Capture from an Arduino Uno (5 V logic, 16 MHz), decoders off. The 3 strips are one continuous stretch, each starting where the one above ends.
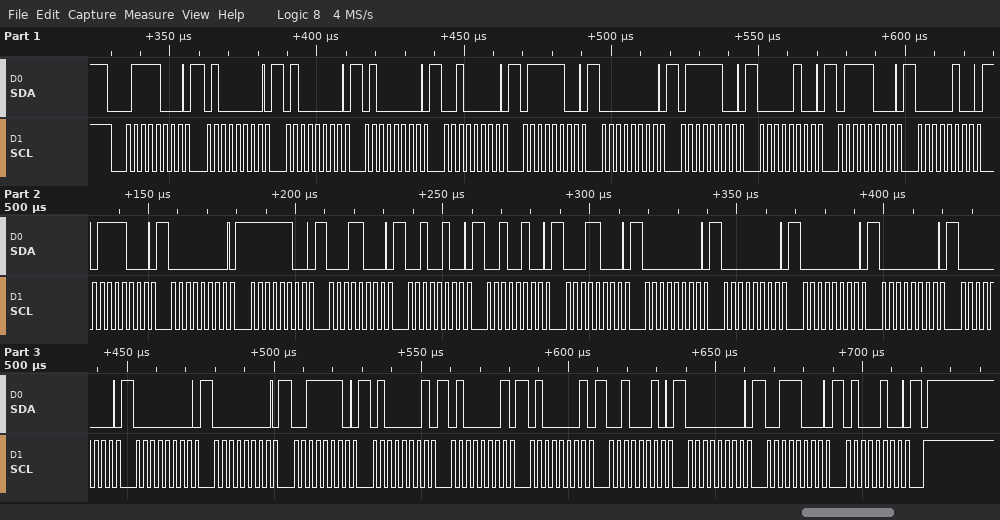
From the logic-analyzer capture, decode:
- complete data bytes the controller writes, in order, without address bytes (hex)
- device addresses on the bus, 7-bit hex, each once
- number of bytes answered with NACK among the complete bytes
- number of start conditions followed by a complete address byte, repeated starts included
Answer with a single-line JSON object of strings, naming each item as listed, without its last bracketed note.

{"complete data bytes the controller writes, in order, without address bytes": "40 40 40 20 7C 00 7C 04 78 04 78 00 FC 18 24 24 18 00 00 00 00 00 00 00 3E 41 41 41 22 00 38 44", "device addresses on the bus, 7-bit hex, each once": "0x3C", "number of bytes answered with NACK among the complete bytes": "0", "number of start conditions followed by a complete address byte, repeated starts included": "1"}
